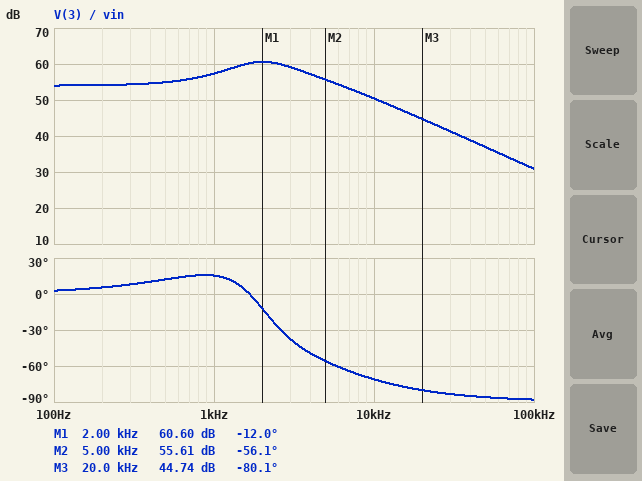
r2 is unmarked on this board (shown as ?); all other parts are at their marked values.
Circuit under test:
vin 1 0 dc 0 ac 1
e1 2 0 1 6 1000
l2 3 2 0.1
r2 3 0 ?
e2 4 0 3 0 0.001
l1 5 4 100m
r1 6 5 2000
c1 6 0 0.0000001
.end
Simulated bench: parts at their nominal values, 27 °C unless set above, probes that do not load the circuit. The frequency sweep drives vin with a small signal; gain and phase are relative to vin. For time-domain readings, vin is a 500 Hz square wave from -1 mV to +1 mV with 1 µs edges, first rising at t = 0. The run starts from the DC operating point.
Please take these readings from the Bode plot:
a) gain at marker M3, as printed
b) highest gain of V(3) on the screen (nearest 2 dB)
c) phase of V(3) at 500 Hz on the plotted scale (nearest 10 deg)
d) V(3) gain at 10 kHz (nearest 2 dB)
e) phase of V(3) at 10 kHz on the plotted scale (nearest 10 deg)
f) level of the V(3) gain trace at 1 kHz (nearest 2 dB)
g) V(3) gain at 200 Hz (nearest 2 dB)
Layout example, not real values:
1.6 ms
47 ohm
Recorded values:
44.74 dB
60 dB
10 deg
50 dB
-70 deg
58 dB
54 dB
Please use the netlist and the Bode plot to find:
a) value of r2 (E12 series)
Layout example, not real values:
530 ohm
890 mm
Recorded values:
2.2 kΩ
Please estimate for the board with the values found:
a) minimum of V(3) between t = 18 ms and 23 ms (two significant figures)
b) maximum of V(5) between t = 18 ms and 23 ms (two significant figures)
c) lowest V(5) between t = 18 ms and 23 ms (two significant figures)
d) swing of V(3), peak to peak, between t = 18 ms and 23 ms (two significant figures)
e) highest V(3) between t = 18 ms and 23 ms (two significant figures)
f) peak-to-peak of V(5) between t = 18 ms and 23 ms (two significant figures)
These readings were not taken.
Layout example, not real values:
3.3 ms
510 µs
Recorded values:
-1.2 V
1.3 mV
-1.3 mV
2.3 V
1.2 V
2.5 mV
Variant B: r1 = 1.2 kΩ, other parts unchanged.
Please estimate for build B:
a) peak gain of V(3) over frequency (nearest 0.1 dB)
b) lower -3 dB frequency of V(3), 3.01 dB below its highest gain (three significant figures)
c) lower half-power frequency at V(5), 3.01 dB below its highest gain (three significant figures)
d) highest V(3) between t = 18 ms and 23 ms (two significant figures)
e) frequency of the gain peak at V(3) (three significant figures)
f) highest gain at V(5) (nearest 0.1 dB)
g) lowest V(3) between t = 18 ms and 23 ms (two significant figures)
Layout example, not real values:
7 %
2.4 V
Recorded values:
62.4 dB
1.59 kHz
1.38 kHz
1.1 V
2.14 kHz
3.2 dB
-1.1 V
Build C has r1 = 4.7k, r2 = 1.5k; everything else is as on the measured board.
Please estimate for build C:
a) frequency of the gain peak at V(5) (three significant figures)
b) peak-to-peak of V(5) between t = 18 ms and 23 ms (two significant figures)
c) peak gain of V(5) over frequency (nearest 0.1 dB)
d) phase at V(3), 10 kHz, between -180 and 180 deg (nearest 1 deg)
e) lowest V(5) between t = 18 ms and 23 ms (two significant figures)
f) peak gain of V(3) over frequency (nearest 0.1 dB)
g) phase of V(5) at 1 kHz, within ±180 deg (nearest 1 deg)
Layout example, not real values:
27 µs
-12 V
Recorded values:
1.16 kHz
2.4 mV
-0.2 dB
-77 deg
-1.2 mV
59.5 dB
-12 deg
